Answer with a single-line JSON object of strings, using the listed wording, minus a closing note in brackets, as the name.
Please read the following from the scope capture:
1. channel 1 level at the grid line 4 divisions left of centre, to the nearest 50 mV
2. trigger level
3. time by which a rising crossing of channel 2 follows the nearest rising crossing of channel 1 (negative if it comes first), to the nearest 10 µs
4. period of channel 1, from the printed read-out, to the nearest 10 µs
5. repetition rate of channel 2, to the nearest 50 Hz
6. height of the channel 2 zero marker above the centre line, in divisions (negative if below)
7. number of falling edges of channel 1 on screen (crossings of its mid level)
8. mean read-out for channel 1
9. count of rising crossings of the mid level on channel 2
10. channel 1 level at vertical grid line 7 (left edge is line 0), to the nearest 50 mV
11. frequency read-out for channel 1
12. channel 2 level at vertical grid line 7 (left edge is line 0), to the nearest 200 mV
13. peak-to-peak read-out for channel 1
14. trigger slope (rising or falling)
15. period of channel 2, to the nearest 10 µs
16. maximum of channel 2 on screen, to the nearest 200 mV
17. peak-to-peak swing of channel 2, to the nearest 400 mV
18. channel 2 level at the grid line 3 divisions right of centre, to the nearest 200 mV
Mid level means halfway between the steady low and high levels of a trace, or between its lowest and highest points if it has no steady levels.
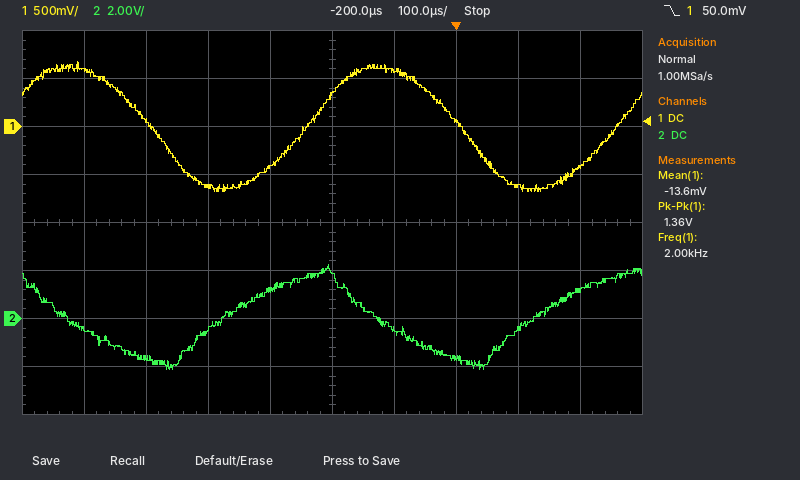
{"channel 1 level at the grid line 4 divisions left of centre, to the nearest 50 mV": "600 mV", "trigger level": "50.0 mV", "time by which a rising crossing of channel 2 follows the nearest rising crossing of channel 1 (negative if it comes first), to the nearest 10 µs": "-130 µs", "period of channel 1, from the printed read-out, to the nearest 10 µs": "500 µs", "repetition rate of channel 2, to the nearest 50 Hz": "2.00 kHz", "height of the channel 2 zero marker above the centre line, in divisions": "-2.0 div", "number of falling edges of channel 1 on screen": "2", "mean read-out for channel 1": "-13.6 mV", "count of rising crossings of the mid level on channel 2": "2", "channel 1 level at vertical grid line 7 (left edge is line 0), to the nearest 50 mV": "50 mV", "frequency read-out for channel 1": "2.00 kHz", "channel 2 level at vertical grid line 7 (left edge is line 0), to the nearest 200 mV": "-1.6 V", "peak-to-peak read-out for channel 1": "1.36 V", "trigger slope": "falling", "period of channel 2, to the nearest 10 µs": "500 µs", "maximum of channel 2 on screen, to the nearest 200 mV": "2.2 V", "peak-to-peak swing of channel 2, to the nearest 400 mV": "4.4 V", "channel 2 level at the grid line 3 divisions right of centre, to the nearest 200 mV": "-400 mV"}
